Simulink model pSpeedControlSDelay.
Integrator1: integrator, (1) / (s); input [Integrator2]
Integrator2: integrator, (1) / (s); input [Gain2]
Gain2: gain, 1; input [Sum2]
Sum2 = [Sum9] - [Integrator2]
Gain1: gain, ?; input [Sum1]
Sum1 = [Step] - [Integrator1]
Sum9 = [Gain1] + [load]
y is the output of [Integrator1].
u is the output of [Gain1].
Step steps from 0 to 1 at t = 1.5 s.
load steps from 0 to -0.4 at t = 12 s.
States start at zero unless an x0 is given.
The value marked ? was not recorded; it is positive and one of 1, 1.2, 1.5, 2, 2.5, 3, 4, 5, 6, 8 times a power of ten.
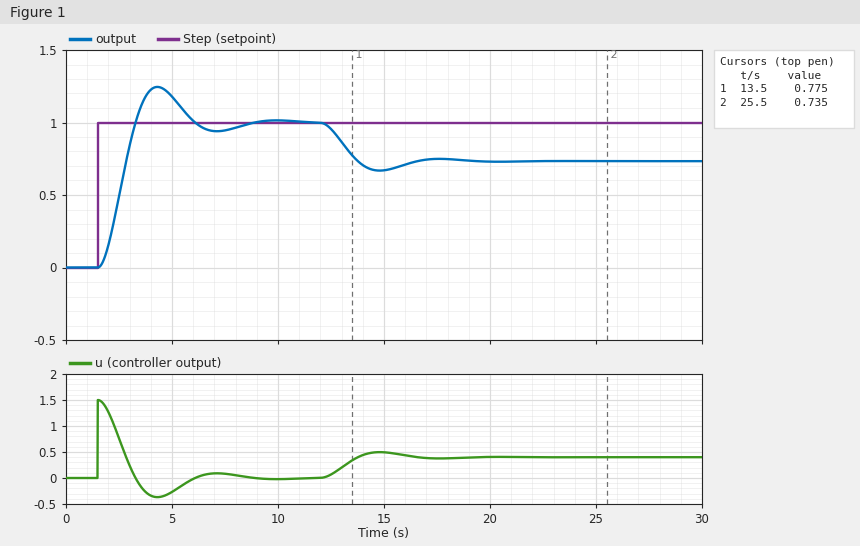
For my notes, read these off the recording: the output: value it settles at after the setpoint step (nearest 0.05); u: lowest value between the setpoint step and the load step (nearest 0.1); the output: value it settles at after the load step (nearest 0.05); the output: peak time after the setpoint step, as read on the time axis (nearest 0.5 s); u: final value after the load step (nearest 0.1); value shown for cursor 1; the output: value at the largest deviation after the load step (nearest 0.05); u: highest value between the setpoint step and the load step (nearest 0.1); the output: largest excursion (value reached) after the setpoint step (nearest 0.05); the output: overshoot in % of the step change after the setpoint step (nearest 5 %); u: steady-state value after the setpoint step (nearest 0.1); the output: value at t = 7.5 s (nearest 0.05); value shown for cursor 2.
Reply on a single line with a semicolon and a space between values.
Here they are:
1.00; -0.4; 0.75; 4.5 s; 0.4; 0.775; 0.65; 1.5; 1.25; 25 %; 0.0; 0.95; 0.735
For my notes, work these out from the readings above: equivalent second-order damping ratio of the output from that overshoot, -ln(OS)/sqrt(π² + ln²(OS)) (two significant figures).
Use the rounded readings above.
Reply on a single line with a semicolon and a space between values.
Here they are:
0.40
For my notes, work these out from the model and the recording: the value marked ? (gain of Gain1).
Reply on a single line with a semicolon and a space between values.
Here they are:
1.5
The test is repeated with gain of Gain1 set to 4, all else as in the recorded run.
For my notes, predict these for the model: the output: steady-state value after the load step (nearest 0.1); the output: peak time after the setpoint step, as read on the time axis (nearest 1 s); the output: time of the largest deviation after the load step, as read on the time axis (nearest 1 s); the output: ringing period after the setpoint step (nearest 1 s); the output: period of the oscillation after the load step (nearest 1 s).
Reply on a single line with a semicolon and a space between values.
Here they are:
0.9; 3 s; 14 s; 3 s; 3 s
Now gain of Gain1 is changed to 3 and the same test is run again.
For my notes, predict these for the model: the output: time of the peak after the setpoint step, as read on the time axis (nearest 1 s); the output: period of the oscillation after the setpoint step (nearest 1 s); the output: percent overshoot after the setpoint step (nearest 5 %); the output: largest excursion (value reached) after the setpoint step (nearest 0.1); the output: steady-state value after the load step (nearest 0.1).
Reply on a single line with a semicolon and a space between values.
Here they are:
3 s; 4 s; 40 %; 1.4; 0.9
